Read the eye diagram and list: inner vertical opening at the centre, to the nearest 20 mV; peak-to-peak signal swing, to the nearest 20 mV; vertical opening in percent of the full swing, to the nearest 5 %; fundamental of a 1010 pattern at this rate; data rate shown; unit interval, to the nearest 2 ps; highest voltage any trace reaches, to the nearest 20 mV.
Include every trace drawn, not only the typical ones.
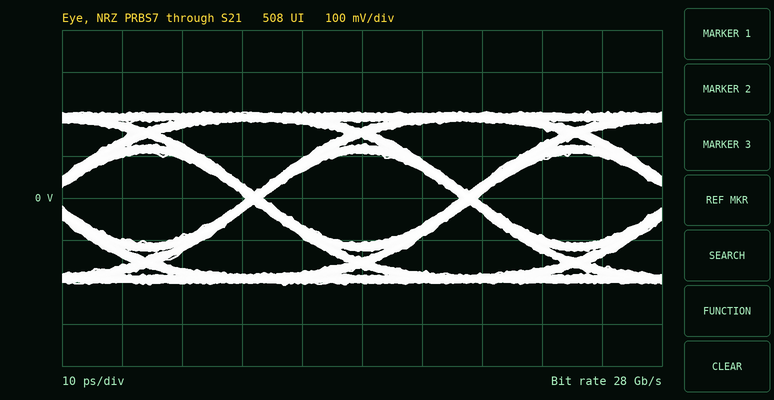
220 mV
420 mV
50 %
14 GHz
28 Gb/s
36 ps
200 mV
